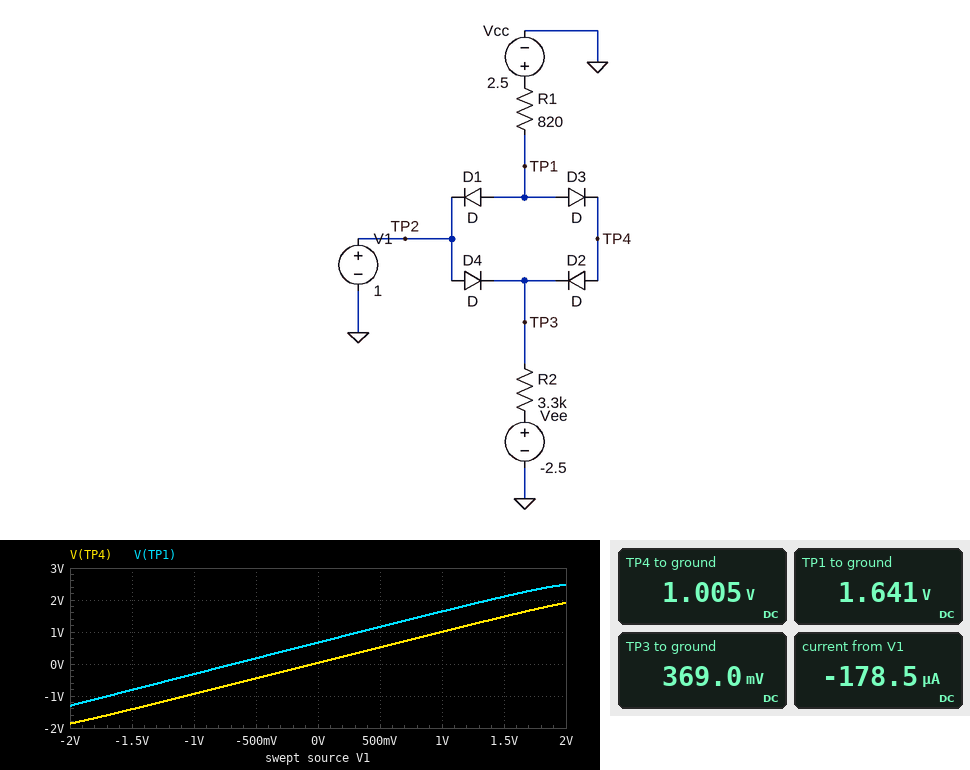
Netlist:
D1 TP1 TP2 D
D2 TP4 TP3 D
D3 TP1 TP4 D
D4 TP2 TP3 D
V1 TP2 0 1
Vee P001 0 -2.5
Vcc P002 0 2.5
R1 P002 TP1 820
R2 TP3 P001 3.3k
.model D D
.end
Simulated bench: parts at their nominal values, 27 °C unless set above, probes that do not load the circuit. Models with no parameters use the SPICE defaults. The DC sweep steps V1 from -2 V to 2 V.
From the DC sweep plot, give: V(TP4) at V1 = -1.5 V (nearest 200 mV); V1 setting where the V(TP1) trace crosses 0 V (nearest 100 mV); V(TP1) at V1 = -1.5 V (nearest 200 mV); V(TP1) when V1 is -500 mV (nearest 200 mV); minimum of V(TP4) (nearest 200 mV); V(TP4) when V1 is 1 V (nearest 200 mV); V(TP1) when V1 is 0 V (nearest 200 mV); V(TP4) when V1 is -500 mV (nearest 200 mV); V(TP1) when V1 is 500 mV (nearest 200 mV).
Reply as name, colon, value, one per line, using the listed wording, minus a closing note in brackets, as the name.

V(TP4) at V1 = -1.5 V: -1.4 V
V1 setting where the V(TP1) trace crosses 0 V: -700 mV
V(TP1) at V1 = -1.5 V: -800 mV
V(TP1) when V1 is -500 mV: 200 mV
minimum of V(TP4): -1.8 V
V(TP4) when V1 is 1 V: 1.0 V
V(TP1) when V1 is 0 V: 600 mV
V(TP4) when V1 is -500 mV: -400 mV
V(TP1) when V1 is 500 mV: 1.2 V
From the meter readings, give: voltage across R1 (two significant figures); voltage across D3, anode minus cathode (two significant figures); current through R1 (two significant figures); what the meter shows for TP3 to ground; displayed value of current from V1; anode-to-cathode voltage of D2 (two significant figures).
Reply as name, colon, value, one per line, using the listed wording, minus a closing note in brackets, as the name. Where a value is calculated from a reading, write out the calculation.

voltage across R1: 2.5 V - 1.641 V = 860 mV
voltage across D3, anode minus cathode: 1.641 V - 1.005 V = 640 mV
current through R1: (2.5 V - 1.641 V) / 820 Ω = 1.0 mA
what the meter shows for TP3 to ground: 369.0 mV
displayed value of current from V1: -178.5 µA
anode-to-cathode voltage of D2: 1.005 V - 369 mV = 640 mV
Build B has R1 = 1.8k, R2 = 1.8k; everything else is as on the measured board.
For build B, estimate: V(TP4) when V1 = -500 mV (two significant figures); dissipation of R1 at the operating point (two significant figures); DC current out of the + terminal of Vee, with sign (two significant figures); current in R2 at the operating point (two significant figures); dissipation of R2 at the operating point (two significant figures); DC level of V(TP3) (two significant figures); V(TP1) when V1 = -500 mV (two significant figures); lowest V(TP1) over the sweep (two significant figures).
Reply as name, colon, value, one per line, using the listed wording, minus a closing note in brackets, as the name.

V(TP4) when V1 = -500 mV: -490 mV
dissipation of R1 at the operating point: 450 µW
DC current out of the + terminal of Vee, with sign: -1.6 mA
current in R2 at the operating point: 1.6 mA
dissipation of R2 at the operating point: 4.5 mW
DC level of V(TP3): 340 mV
V(TP1) when V1 = -500 mV: 150 mV
lowest V(TP1) over the sweep: -1.3 V
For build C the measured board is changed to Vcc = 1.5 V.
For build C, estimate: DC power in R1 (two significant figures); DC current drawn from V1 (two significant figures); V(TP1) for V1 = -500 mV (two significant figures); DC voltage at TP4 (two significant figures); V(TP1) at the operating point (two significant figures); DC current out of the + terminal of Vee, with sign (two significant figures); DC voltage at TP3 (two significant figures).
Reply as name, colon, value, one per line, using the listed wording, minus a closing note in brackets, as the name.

DC power in R1: 710 nW
DC current drawn from V1: 830 µA
V(TP1) for V1 = -500 mV: 160 mV
DC voltage at TP4: 910 mV
V(TP1) at the operating point: 1.5 V
DC current out of the + terminal of Vee, with sign: -860 µA
DC voltage at TP3: 350 mV
